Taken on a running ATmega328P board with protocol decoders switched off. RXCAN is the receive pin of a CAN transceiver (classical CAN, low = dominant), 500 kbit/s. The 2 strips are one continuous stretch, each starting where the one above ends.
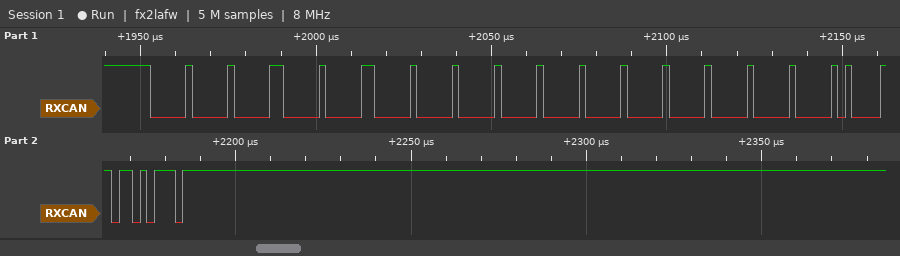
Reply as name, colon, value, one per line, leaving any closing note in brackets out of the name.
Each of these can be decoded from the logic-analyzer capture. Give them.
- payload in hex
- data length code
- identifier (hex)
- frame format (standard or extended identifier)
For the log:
payload in hex: 01 00 00 00 00 00 00 00
data length code: 8
identifier: 0x000
frame format: standard
